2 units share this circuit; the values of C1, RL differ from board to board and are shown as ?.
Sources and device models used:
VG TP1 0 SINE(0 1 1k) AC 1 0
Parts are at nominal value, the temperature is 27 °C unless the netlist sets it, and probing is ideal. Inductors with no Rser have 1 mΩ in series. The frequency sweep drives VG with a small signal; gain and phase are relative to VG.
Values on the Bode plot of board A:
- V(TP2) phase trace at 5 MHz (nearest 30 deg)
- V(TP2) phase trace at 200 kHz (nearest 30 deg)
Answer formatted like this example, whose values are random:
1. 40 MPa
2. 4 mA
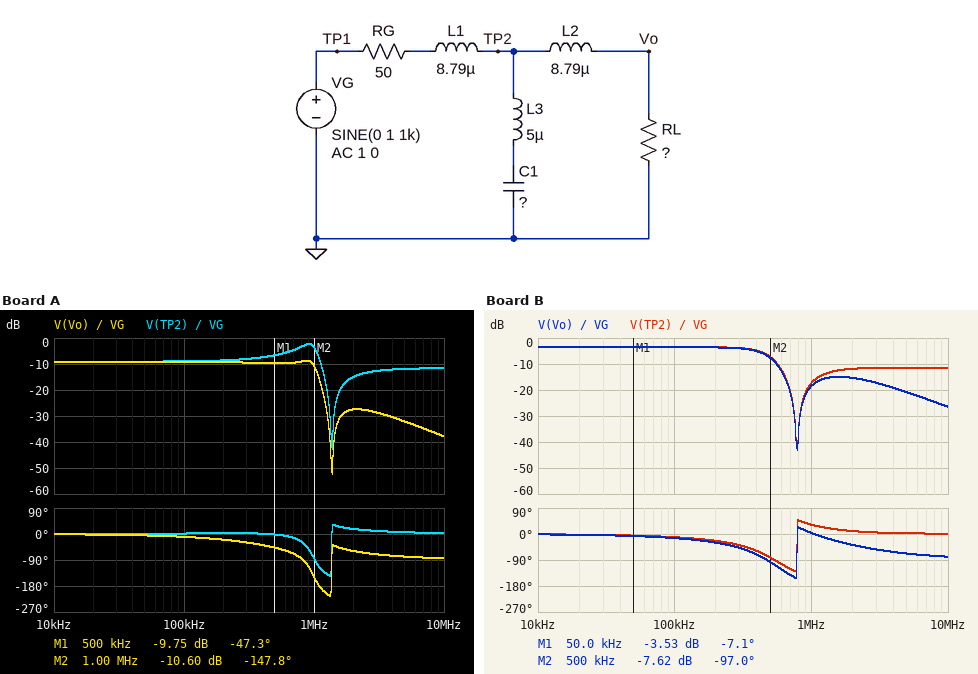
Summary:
1. 0 deg
2. 0 deg
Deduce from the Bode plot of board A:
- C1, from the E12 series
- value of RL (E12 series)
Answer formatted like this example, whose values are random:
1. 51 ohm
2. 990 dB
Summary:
1. 2.7 nF
2. 27 Ω
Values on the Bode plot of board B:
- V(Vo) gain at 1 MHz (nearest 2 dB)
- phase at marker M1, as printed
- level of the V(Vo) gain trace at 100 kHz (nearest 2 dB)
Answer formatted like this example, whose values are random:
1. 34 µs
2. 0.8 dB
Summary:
1. -18 dB
2. -7.1 deg
3. -4 dB
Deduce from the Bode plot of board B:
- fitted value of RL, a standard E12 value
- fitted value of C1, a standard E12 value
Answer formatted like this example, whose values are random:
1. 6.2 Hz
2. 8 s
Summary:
1. 100 Ω
2. 8.2 nF
